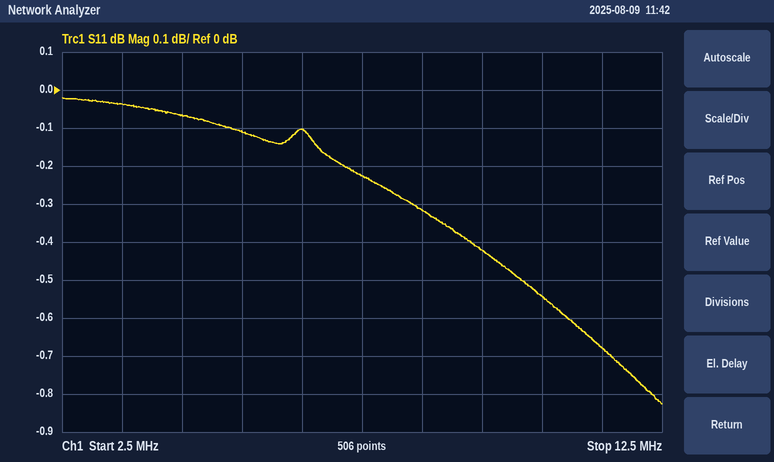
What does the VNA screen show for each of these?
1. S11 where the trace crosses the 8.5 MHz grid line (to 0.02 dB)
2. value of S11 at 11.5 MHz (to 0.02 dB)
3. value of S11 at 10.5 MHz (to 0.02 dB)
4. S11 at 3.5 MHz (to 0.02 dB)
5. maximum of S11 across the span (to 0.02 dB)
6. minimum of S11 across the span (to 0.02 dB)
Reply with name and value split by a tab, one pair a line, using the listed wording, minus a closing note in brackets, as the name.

S11 where the trace crosses the 8.5 MHz grid line	-0.32 dB
value of S11 at 11.5 MHz	-0.68 dB
value of S11 at 10.5 MHz	-0.54 dB
S11 at 3.5 MHz	-0.04 dB
maximum of S11 across the span	-0.02 dB
minimum of S11 across the span	-0.82 dB
